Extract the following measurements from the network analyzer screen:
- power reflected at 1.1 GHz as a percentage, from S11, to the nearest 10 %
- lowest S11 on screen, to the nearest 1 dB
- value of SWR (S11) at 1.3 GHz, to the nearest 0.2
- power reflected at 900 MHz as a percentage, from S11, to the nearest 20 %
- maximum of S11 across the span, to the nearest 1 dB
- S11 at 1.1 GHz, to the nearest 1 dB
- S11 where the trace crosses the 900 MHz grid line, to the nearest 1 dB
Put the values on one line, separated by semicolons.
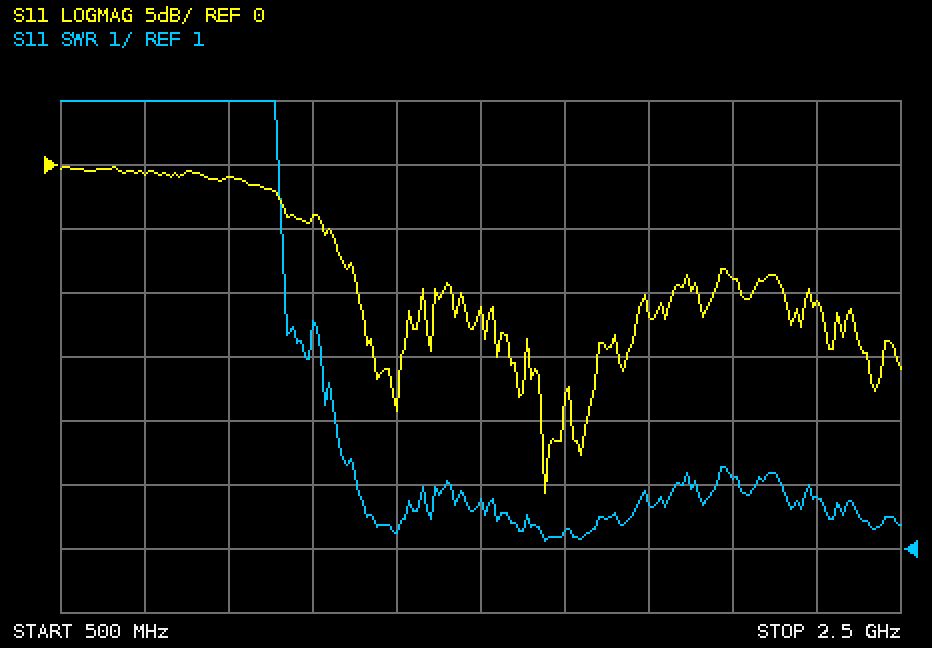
40 %; -26 dB; 1.2; 80 %; 0 dB; -4 dB; -1 dB
